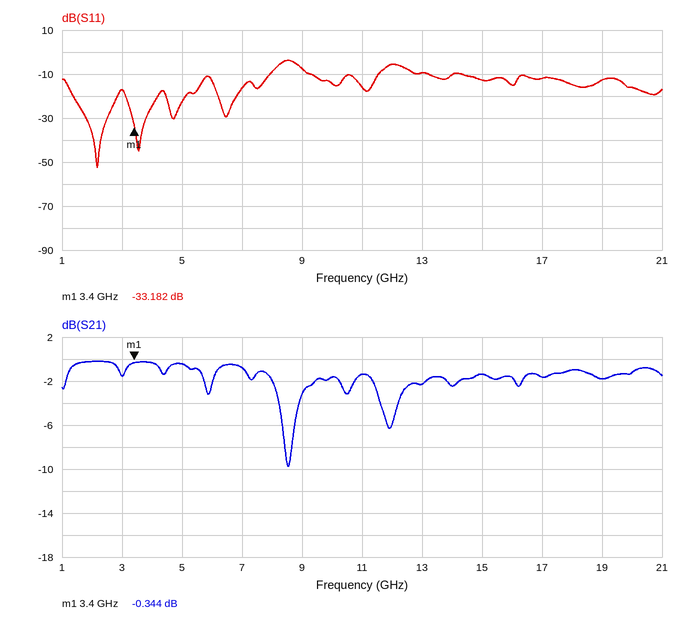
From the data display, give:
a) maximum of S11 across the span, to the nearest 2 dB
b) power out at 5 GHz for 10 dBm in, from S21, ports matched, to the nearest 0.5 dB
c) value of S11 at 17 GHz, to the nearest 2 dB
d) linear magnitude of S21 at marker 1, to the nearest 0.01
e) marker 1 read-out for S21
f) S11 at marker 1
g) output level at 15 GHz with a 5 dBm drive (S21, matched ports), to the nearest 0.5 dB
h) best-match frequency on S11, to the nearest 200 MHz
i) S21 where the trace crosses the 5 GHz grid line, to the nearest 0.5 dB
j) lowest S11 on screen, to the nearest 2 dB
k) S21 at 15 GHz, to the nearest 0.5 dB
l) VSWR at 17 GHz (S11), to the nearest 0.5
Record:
-4 dB
9.5 dBm
-12 dB
0.96
-0.344 dB
-33.182 dB
3.5 dBm
2.2 GHz
-0.5 dB
-52 dB
-1.5 dB
1.5
